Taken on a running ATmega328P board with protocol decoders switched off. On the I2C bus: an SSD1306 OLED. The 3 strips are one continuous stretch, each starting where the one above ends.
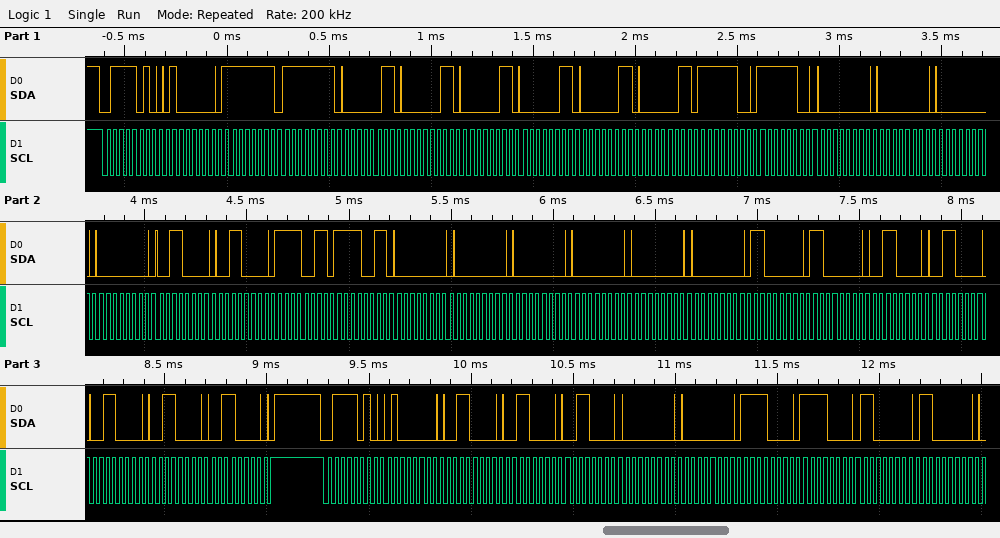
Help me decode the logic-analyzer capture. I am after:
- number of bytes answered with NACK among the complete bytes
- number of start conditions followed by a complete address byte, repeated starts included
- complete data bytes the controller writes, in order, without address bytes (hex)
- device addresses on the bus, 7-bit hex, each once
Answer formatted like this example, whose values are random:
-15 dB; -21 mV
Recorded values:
0; 2; 40 FF FF 03 03 03 03 03 03 FC FC 00 00 00 00 30 30 F3 F3 00 00 00 00 00 00 C0 C0 30 30 30 30 30 40 30 30 30 00 00 F0 F0 C0 C0; 0x3D
